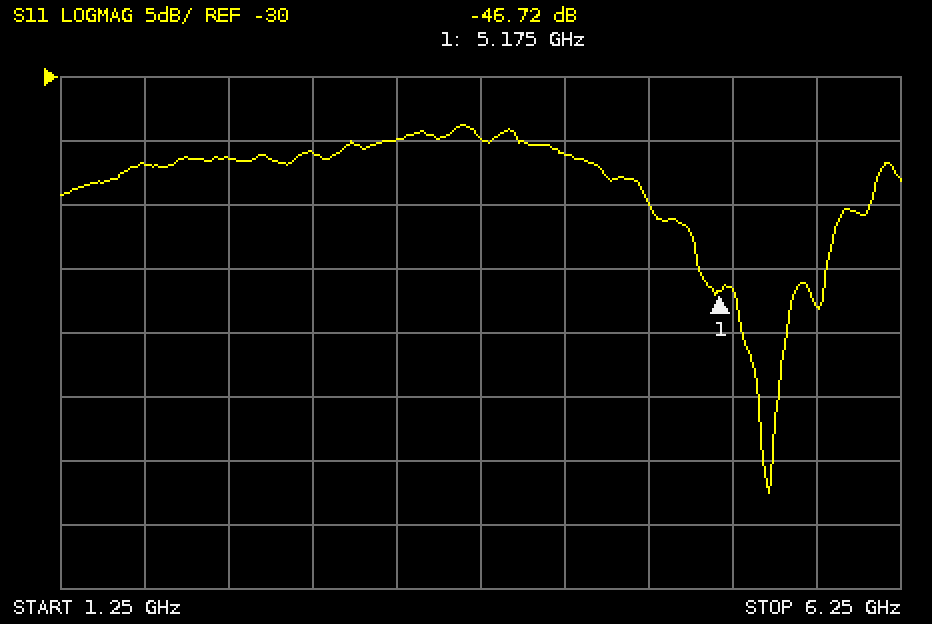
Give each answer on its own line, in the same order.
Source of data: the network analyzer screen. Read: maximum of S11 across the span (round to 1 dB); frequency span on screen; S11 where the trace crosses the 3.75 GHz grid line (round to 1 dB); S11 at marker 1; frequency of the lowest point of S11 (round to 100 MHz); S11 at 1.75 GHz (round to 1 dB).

-34 dB
5 GHz
-35 dB
-46.72 dB
5.5 GHz
-37 dB
